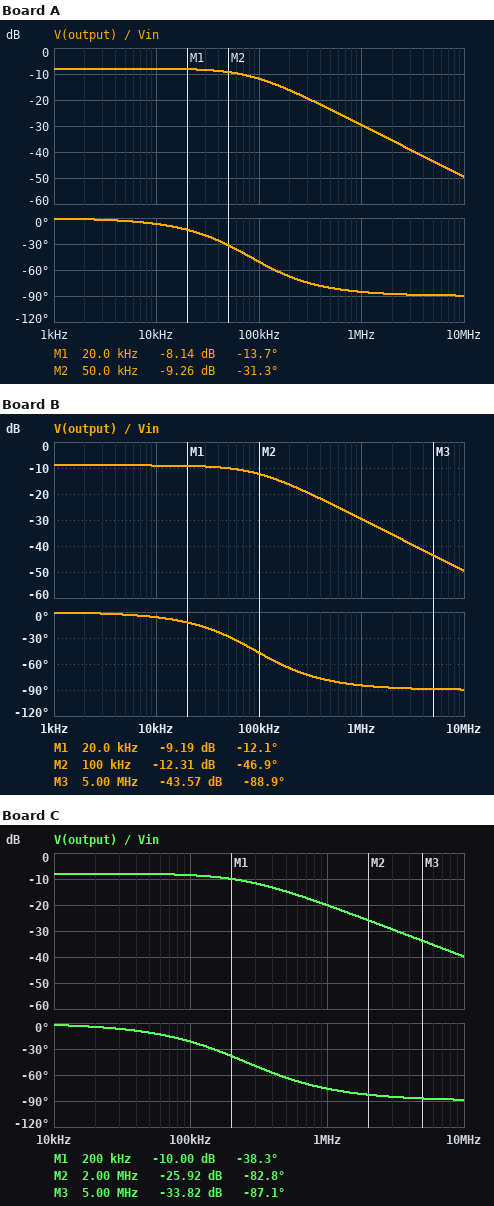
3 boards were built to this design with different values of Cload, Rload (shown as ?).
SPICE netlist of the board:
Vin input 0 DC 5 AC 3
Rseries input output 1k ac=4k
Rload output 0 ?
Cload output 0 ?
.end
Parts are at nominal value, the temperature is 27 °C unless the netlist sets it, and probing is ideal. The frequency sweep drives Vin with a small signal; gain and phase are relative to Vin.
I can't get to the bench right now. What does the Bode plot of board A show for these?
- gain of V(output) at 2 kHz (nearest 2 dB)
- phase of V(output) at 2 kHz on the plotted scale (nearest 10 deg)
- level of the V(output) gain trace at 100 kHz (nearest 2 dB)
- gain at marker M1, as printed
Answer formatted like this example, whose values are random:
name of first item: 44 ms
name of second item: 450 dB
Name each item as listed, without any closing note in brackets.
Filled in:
gain of V(output) at 2 kHz: -8 dB
phase of V(output) at 2 kHz on the plotted scale: 0 deg
level of the V(output) gain trace at 100 kHz: -12 dB
gain at marker M1, as printed: -8.14 dB
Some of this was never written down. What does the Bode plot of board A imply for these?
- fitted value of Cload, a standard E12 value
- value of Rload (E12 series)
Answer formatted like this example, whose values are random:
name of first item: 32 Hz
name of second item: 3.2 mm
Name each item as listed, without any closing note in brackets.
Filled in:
fitted value of Cload, a standard E12 value: 1.2 nF
value of Rload: 2.7 kΩ
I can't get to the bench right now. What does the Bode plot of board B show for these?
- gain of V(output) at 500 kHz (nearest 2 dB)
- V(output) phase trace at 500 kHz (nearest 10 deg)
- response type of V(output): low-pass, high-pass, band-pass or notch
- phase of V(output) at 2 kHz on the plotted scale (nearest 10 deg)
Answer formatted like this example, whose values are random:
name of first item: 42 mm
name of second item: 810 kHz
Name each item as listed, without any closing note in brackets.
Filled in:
gain of V(output) at 500 kHz: -24 dB
V(output) phase trace at 500 kHz: -80 deg
response type of V(output): low-pass, high-pass, band-pass or notch: low-pass
phase of V(output) at 2 kHz on the plotted scale: 0 deg
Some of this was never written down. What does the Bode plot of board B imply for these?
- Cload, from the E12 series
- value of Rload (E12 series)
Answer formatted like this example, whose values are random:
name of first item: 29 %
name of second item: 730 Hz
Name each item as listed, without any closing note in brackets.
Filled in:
Cload, from the E12 series: 1.2 nF
value of Rload: 2.2 kΩ
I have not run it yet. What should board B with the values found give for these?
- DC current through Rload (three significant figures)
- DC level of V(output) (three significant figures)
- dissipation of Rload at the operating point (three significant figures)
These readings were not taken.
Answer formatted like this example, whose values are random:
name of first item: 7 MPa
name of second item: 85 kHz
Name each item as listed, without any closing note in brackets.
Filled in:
DC current through Rload: 1.56 mA
DC level of V(output): 3.44 V
dissipation of Rload at the operating point: 5.37 mW
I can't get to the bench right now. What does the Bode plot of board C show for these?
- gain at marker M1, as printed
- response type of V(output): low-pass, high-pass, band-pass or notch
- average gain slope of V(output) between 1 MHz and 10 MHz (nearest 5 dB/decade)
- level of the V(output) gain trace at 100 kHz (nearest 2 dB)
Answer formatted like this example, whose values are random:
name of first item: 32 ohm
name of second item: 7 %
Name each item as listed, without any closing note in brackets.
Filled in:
gain at marker M1, as printed: -10.00 dB
response type of V(output): low-pass, high-pass, band-pass or notch: low-pass
average gain slope of V(output) between 1 MHz and 10 MHz: -20 dB/decade
level of the V(output) gain trace at 100 kHz: -8 dB
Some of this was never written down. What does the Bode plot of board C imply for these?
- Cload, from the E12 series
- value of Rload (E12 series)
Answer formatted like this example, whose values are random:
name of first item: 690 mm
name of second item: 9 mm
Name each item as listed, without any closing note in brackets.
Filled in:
Cload, from the E12 series: 390 pF
value of Rload: 2.7 kΩ
